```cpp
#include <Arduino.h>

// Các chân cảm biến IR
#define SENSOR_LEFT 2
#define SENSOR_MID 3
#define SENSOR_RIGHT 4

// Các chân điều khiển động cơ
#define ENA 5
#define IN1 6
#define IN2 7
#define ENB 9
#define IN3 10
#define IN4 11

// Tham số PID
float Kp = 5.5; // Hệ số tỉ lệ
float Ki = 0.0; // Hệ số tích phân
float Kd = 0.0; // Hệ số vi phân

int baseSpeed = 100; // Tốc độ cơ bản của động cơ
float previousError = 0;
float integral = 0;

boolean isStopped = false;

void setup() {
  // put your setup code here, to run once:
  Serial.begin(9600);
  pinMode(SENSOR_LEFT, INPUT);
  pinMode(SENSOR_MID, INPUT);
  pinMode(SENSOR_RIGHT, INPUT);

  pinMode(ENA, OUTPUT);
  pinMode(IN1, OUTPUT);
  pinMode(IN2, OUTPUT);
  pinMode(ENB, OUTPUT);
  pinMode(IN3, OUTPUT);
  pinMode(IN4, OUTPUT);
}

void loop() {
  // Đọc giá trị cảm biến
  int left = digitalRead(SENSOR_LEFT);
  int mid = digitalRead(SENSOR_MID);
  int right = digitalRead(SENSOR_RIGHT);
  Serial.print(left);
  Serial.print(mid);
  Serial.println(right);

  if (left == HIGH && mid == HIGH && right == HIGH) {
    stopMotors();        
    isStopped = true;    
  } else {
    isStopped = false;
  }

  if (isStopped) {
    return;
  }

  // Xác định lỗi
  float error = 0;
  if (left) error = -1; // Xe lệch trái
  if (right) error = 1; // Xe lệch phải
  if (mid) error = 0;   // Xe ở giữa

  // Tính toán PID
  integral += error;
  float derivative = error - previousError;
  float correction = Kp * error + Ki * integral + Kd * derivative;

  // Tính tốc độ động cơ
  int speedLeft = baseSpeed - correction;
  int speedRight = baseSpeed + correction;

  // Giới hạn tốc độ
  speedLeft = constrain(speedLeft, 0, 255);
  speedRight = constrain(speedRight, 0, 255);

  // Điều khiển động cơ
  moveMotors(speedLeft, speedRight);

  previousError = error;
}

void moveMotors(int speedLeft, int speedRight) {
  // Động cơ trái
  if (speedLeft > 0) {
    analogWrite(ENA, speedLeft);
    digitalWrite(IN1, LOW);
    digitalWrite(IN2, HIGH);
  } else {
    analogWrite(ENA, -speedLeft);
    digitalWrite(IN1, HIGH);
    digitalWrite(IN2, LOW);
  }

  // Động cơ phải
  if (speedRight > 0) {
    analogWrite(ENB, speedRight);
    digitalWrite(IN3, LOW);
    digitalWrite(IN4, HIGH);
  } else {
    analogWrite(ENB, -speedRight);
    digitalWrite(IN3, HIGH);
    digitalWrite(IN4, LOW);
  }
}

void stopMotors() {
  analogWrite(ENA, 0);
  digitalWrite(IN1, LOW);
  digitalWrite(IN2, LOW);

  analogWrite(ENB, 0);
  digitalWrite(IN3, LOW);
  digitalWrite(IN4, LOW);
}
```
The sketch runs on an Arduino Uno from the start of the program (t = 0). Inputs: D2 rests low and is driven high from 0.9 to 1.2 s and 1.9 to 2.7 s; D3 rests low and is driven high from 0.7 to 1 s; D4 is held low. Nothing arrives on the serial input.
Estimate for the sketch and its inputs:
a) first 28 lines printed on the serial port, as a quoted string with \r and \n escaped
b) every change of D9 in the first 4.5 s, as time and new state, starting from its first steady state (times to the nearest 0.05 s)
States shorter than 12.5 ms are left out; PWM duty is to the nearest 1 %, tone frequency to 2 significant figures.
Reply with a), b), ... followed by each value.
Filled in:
a) "000\r\n000\r\n000\r\n000\r\n000\r\n000\r\n000\r\n000\r\n000\r\n000\r\n000\r\n000\r\n000\r\n000\r\n000\r\n000\r\n000\r\n000\r\n000\r\n000\r\n000\r\n000\r\n000\r\n000\r\n000\r\n000\r\n000\r\n000\r\n"
b) 0 s PWM 39 %; 1 s PWM 37 %; 1.2 s PWM 39 %; 1.9 s PWM 37 %; 2.7 s PWM 39 %
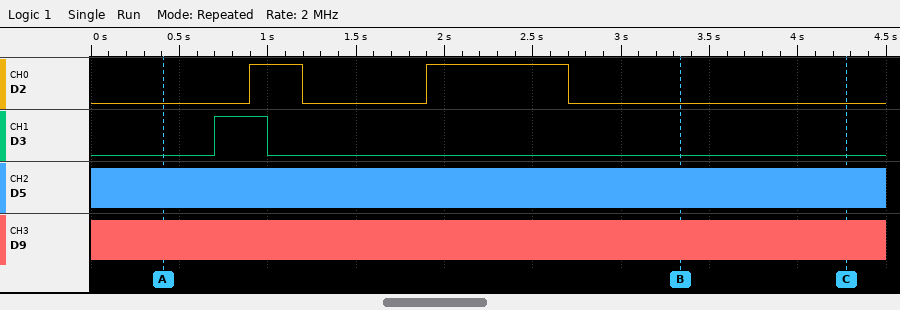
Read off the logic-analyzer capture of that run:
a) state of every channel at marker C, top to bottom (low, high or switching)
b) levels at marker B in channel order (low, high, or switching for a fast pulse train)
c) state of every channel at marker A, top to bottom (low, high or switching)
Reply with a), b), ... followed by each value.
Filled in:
a) D2 low, D3 low, D5 switching, D9 switching
b) D2 low, D3 low, D5 switching, D9 switching
c) D2 low, D3 low, D5 switching, D9 switching
